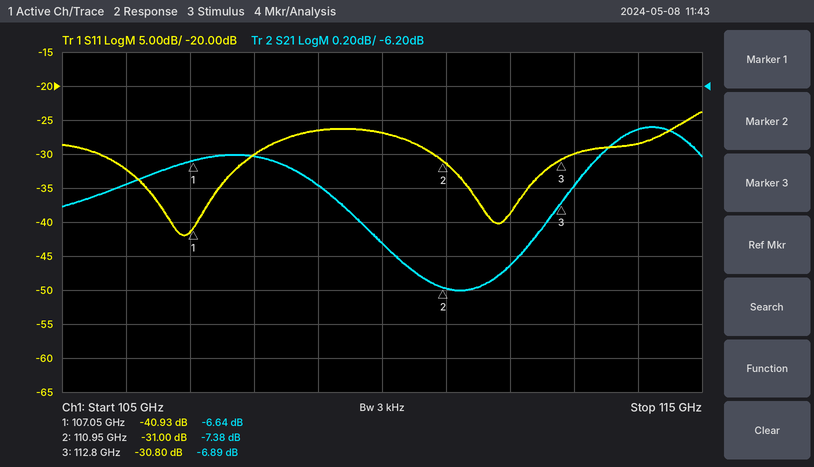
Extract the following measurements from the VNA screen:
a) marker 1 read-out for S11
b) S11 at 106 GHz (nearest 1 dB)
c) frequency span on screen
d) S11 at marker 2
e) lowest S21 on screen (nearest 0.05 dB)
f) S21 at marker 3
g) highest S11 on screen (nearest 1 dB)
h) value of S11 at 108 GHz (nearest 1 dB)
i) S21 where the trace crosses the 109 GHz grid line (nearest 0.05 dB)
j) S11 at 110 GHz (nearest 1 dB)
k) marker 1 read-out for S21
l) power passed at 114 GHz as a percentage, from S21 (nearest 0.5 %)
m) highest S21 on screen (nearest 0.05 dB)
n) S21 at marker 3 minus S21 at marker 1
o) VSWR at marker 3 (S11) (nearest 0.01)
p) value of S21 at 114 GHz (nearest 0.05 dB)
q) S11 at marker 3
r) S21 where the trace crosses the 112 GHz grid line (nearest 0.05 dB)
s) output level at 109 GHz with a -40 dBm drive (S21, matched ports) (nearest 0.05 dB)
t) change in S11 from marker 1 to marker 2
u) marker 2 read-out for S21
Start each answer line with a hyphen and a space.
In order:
- -40.93 dB
- -32 dB
- 10 GHz
- -31.00 dB
- -7.40 dB
- -6.89 dB
- -24 dB
- -30 dB
- -6.80 dB
- -27 dB
- -6.64 dB
- 22.5 %
- -6.45 dB
- -0.25 dB
- 1.06
- -6.45 dB
- -30.80 dB
- -7.25 dB
- -46.80 dBm
- 9.93 dB
- -7.38 dB
